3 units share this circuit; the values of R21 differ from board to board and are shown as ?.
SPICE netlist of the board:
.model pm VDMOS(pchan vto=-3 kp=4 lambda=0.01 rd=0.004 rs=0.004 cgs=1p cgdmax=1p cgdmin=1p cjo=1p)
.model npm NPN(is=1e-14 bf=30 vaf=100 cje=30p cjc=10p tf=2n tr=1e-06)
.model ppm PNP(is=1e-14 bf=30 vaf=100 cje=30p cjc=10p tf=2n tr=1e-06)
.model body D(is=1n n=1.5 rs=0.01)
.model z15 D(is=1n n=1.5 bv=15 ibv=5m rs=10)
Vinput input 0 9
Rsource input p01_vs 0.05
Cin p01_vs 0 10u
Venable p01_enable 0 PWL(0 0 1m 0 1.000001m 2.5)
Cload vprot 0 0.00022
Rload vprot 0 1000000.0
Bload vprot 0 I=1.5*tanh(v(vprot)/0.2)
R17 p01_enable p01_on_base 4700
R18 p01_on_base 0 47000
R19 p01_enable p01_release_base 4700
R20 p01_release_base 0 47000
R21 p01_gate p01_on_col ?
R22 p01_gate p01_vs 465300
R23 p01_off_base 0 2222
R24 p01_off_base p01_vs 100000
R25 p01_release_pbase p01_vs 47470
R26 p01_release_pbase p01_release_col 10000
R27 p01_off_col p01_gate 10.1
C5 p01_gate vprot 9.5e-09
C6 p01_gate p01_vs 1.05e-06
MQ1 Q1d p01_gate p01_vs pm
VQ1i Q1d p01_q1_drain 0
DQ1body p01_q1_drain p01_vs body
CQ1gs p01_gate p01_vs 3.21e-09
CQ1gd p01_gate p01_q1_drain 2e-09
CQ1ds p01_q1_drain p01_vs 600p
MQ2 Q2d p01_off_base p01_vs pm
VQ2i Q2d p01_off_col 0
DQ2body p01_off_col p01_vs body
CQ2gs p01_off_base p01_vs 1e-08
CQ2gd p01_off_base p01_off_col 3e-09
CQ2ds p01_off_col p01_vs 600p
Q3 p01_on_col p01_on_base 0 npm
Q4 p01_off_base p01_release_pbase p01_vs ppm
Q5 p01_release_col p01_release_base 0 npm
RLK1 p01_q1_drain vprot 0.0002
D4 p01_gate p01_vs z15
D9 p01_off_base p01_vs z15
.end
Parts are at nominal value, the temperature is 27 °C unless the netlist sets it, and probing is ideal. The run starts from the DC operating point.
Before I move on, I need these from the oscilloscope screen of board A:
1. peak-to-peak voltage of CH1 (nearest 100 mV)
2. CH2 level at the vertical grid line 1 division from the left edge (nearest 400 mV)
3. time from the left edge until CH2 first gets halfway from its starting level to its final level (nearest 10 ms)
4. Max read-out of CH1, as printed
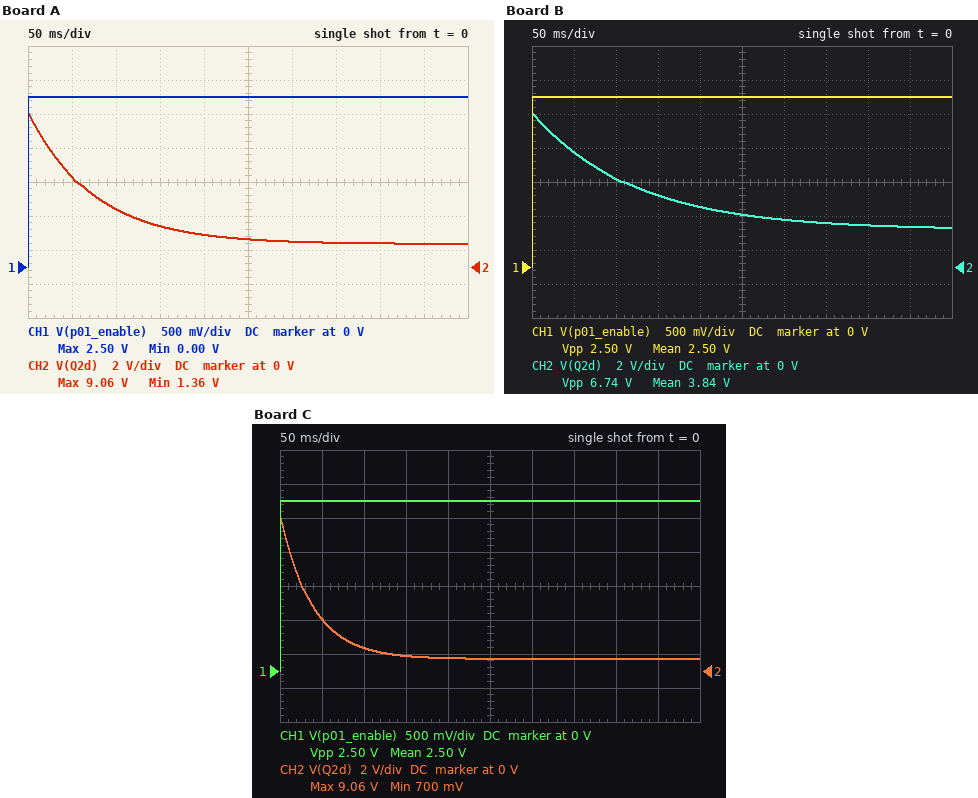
2.5 V
5.2 V
50 ms
2.50 V
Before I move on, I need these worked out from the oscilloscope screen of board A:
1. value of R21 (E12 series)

82 kΩ
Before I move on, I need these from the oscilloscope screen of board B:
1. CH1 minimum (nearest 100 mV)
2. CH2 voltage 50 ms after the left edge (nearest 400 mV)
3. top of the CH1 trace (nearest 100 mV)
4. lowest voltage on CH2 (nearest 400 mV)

0 V
6.8 V
2.5 V
2.4 V
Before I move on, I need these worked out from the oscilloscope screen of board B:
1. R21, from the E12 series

150 kΩ
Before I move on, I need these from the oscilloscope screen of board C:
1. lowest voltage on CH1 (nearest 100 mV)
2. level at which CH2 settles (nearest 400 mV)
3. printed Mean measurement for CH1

0 V
800 mV
2.50 V
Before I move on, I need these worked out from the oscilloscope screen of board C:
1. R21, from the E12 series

39 kΩ
